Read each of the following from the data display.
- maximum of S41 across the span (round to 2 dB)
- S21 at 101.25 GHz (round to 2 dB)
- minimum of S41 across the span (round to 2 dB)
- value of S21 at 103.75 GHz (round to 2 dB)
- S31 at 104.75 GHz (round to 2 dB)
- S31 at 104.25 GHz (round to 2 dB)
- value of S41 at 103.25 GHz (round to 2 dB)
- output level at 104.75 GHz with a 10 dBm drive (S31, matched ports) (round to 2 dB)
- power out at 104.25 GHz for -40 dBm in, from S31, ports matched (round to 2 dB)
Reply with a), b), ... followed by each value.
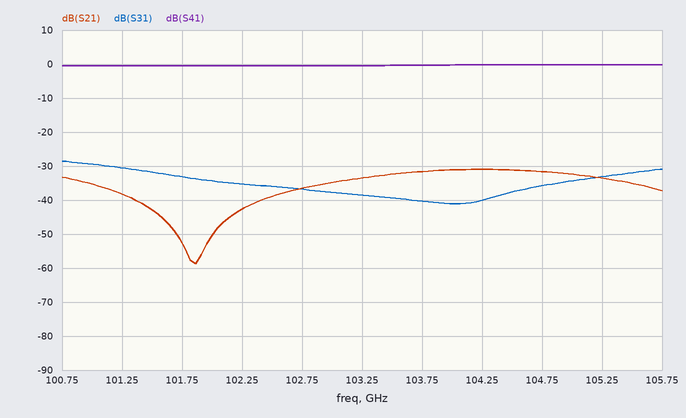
a) 0 dB
b) -38 dB
c) 0 dB
d) -32 dB
e) -36 dB
f) -40 dB
g) 0 dB
h) -26 dBm
i) -80 dBm
